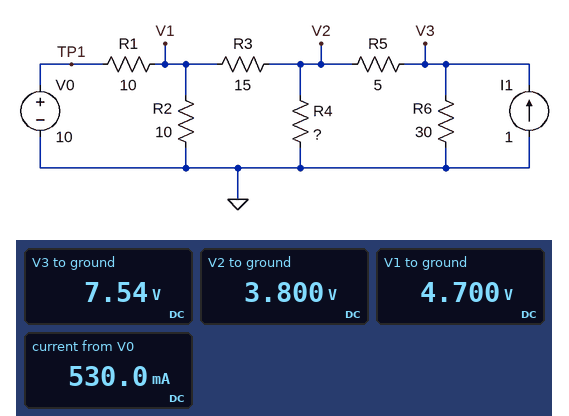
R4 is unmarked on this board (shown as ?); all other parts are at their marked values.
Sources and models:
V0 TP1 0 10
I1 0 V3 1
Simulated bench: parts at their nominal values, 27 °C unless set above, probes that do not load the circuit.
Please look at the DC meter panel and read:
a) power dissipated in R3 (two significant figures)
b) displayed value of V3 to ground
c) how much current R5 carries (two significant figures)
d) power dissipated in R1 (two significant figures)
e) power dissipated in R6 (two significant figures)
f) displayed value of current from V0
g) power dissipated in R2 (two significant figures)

54 mW
7.54 V
750 mA
2.8 W
1.9 W
530.0 mA
2.2 W
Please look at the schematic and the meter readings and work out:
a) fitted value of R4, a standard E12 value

4.7 Ω
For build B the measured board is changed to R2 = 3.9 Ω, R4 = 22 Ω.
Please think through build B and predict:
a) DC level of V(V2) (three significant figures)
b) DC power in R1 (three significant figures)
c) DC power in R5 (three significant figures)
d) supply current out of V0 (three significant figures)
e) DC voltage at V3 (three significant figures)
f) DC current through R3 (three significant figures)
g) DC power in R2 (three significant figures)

7.79 V
4.11 W
2.01 W
641 mA
11.0 V
280 mA
3.31 W
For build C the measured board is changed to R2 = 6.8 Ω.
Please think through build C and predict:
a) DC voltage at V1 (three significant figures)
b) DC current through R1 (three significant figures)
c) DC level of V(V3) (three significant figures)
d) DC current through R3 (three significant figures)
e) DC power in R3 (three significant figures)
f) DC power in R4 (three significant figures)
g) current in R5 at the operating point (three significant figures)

3.96 V
604 mA
7.41 V
21.4 mA
6.86 mW
2.82 W
753 mA
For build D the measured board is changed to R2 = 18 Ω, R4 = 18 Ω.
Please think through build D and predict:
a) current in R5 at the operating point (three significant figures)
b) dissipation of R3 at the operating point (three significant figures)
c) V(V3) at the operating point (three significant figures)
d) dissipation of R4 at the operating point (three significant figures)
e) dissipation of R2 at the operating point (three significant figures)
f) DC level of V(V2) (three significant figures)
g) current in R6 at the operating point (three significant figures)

604 mA
191 mW
11.9 V
4.35 W
2.84 W
8.85 V
396 mA
